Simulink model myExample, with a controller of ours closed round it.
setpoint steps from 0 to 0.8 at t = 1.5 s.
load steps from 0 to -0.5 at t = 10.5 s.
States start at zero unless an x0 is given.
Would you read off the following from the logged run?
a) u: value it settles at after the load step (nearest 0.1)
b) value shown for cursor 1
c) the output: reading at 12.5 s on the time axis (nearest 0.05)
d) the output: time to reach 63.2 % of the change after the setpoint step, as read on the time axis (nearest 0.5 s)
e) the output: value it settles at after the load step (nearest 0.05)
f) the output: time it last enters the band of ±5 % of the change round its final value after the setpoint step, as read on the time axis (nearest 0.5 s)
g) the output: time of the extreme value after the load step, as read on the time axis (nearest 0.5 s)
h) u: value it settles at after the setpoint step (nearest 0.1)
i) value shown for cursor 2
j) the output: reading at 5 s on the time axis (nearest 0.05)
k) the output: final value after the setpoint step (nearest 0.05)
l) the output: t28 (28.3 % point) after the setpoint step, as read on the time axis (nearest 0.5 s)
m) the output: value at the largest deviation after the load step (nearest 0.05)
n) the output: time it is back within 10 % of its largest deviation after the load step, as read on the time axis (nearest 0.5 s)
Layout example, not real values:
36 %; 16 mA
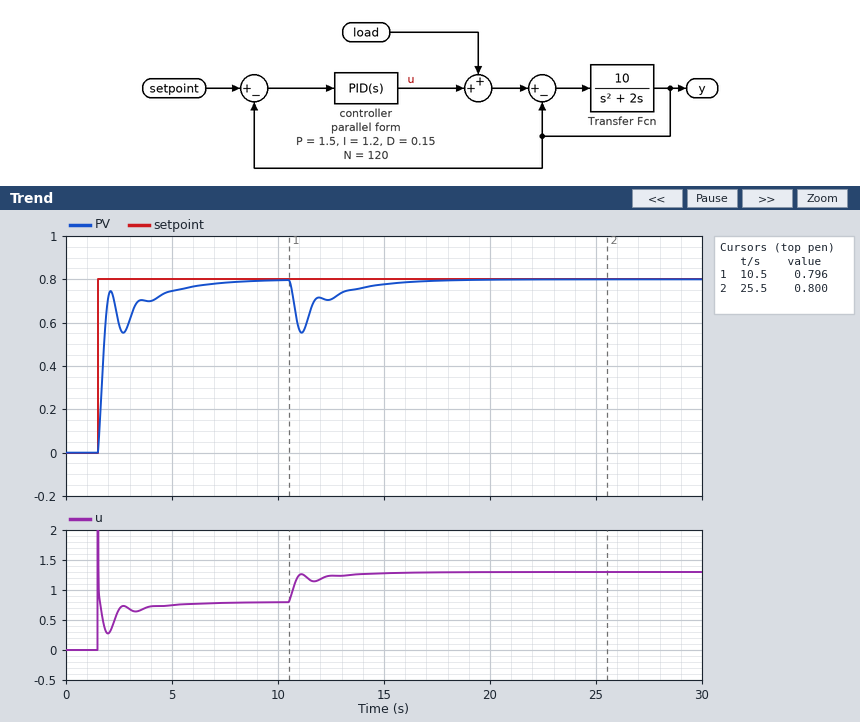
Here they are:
1.3; 0.796; 0.70; 2.0 s; 0.80; 5.5 s; 11.0 s; 0.8; 0.800; 0.75; 0.80; 1.5 s; 0.55; 15.0 s
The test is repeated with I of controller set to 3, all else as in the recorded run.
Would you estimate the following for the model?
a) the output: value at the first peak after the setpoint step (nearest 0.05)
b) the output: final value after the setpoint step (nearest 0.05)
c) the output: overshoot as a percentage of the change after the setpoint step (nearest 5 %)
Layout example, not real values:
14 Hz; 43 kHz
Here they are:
0.90; 0.80; 10 %
